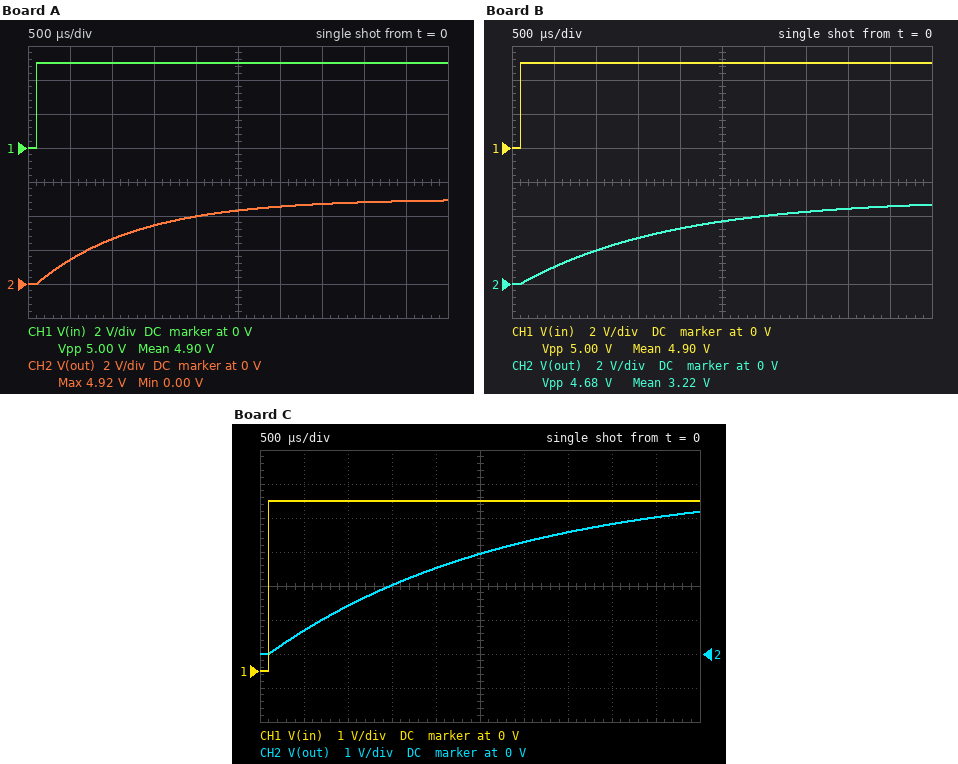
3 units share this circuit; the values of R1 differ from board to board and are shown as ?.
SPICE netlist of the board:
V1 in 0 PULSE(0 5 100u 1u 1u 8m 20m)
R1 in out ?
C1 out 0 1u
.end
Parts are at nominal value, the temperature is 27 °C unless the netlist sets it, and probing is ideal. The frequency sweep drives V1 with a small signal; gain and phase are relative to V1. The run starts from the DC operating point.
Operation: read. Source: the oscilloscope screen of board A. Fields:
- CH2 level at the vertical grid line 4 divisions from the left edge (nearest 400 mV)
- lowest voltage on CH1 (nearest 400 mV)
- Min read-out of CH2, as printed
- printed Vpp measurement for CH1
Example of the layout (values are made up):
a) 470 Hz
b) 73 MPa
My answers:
a) 4.0 V
b) 0 V
c) 0.00 V
d) 5.00 V
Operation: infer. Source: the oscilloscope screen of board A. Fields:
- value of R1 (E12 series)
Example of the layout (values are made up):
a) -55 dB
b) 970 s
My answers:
a) 1.2 kΩ
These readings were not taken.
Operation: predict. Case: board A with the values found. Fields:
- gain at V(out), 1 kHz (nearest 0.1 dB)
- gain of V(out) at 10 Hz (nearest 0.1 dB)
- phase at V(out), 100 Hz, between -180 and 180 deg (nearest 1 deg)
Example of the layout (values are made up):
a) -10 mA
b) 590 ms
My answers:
a) -17.6 dB
b) 0 dB
c) -37 deg
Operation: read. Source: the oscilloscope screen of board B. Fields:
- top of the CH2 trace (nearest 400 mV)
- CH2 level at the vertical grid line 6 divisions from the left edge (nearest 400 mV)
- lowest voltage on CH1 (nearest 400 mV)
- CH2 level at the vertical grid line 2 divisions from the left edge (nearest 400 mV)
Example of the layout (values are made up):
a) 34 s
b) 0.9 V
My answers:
a) 4.8 V
b) 4.0 V
c) 0 V
d) 2.0 V
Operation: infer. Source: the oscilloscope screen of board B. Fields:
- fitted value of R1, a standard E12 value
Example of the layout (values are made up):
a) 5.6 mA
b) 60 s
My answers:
a) 1.8 kΩ
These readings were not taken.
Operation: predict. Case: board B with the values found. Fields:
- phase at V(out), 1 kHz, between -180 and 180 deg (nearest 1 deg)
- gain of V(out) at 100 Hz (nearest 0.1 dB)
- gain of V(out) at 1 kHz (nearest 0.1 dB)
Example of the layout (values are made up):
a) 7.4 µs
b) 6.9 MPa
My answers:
a) -85 deg
b) -3.6 dB
c) -21.1 dB
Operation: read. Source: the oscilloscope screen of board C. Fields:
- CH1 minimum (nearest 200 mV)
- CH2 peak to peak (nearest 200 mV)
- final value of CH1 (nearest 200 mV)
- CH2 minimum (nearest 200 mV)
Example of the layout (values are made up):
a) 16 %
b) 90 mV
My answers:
a) 0 V
b) 4.2 V
c) 5.0 V
d) 0 V
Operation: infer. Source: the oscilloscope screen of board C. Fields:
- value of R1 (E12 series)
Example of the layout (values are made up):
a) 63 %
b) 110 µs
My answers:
a) 2.7 kΩ
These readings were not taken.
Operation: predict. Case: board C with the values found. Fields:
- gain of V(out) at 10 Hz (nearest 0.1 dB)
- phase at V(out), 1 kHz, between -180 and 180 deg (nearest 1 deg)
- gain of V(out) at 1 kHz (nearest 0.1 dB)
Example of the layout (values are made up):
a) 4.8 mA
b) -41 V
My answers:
a) -0.1 dB
b) -87 deg
c) -24.6 dB
